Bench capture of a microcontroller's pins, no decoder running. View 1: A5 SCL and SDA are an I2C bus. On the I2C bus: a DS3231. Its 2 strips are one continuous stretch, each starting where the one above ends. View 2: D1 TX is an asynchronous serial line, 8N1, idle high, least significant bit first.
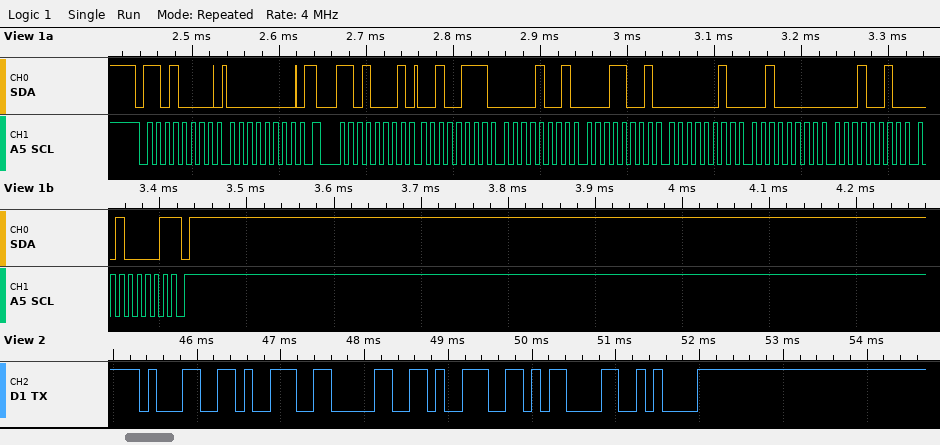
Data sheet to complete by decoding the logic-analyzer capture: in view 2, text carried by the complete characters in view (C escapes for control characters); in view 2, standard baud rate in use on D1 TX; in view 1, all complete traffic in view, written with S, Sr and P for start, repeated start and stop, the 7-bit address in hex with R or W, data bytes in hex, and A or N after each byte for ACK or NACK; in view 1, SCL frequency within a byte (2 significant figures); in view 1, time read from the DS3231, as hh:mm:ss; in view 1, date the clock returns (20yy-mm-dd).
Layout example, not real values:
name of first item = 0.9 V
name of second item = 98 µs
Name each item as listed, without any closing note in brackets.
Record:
in view 2, text carried by the complete characters in view = "1909\r\n"
in view 2, standard baud rate in use on D1 TX = 9600 baud
in view 1, all complete traffic in view, written with S, Sr and P for start, repeated start and stop, the 7-bit address in hex with R or W, data bytes in hex, and A or N after each byte for ACK or NACK = S 68W A 00 A Sr 68R A 27 A 09 A 19 A 02 A 20 A 12 A 21 N P
in view 1, SCL frequency within a byte = 100 kHz
in view 1, time read from the DS3231, as hh:mm:ss = 19:09:27
in view 1, date the clock returns = 2021-12-20
